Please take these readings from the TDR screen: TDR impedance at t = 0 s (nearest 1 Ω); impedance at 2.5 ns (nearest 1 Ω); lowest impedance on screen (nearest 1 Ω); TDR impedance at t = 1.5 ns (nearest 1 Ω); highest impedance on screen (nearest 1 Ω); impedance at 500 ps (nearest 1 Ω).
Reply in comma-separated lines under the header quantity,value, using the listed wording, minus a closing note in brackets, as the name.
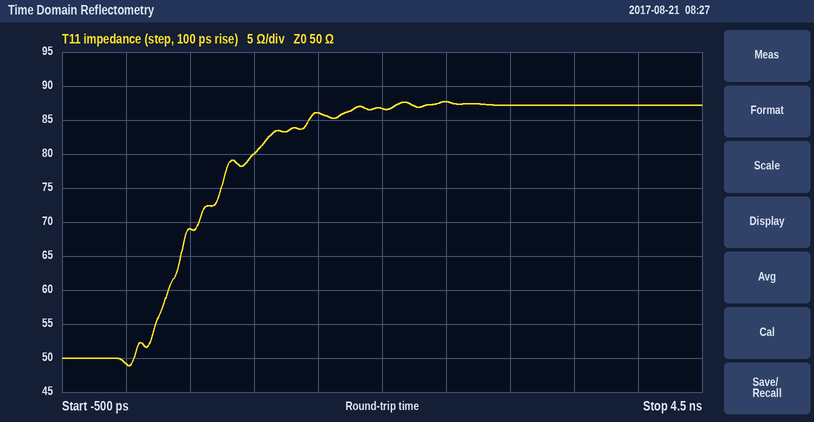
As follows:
quantity,value
TDR impedance at t = 0 s,49 Ω
impedance at 2.5 ns,88 Ω
lowest impedance on screen,49 Ω
TDR impedance at t = 1.5 ns,86 Ω
highest impedance on screen,88 Ω
impedance at 500 ps,69 Ω
